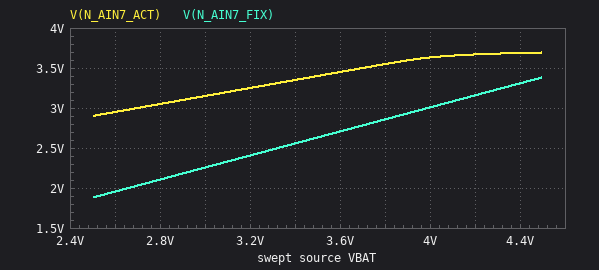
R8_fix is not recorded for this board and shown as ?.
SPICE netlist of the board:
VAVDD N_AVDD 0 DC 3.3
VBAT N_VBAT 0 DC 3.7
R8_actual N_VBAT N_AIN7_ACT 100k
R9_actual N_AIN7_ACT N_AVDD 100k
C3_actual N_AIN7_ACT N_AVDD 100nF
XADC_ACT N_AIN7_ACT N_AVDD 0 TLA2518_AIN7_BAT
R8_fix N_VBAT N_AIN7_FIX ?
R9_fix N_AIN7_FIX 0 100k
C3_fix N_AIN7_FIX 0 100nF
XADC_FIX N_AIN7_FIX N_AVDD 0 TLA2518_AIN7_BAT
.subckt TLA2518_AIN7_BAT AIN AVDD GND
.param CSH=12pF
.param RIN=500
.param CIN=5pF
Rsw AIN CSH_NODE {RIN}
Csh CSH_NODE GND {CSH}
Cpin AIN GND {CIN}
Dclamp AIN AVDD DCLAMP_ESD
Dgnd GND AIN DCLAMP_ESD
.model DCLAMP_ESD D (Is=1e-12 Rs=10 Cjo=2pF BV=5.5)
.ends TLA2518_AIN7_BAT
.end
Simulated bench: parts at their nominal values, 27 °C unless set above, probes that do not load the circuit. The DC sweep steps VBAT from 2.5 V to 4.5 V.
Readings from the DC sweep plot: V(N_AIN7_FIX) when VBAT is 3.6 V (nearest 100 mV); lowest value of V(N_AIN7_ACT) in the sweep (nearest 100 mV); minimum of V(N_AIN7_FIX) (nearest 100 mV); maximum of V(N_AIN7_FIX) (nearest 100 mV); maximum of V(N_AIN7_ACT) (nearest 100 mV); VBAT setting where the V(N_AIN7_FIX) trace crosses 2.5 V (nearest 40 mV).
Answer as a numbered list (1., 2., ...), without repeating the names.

1. 2.7 V
2. 2.9 V
3. 1.9 V
4. 3.4 V
5. 3.7 V
6. 3.32 V
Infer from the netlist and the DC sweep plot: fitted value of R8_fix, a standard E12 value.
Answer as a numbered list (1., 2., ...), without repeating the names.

1. 33 kΩ
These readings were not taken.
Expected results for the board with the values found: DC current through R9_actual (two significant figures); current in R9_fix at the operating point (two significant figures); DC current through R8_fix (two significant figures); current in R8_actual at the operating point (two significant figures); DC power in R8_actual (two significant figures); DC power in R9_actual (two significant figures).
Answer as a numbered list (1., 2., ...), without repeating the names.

1. 2.0 µA
2. 28 µA
3. 28 µA
4. 2.0 µA
5. 400 nW
6. 400 nW
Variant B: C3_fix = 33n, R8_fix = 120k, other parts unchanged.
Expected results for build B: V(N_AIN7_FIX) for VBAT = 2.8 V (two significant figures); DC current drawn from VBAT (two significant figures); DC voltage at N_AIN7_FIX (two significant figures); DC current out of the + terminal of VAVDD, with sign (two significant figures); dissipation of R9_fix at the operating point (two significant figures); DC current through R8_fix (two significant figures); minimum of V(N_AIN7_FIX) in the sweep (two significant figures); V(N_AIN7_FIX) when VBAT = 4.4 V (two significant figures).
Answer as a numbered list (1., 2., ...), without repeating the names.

1. 1.3 V
2. 19 µA
3. 1.7 V
4. -2.0 µA
5. 28 µW
6. 17 µA
7. 1.1 V
8. 2.0 V
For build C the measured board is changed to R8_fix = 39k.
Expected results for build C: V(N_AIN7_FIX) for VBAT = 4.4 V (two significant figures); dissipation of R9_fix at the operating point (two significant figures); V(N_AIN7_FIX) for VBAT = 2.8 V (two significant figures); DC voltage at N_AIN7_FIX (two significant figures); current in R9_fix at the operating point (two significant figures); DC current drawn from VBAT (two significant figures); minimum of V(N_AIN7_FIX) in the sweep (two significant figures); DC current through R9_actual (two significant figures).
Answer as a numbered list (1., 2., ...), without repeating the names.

1. 3.2 V
2. 71 µW
3. 2.0 V
4. 2.7 V
5. 27 µA
6. 29 µA
7. 1.8 V
8. 2.0 µA
